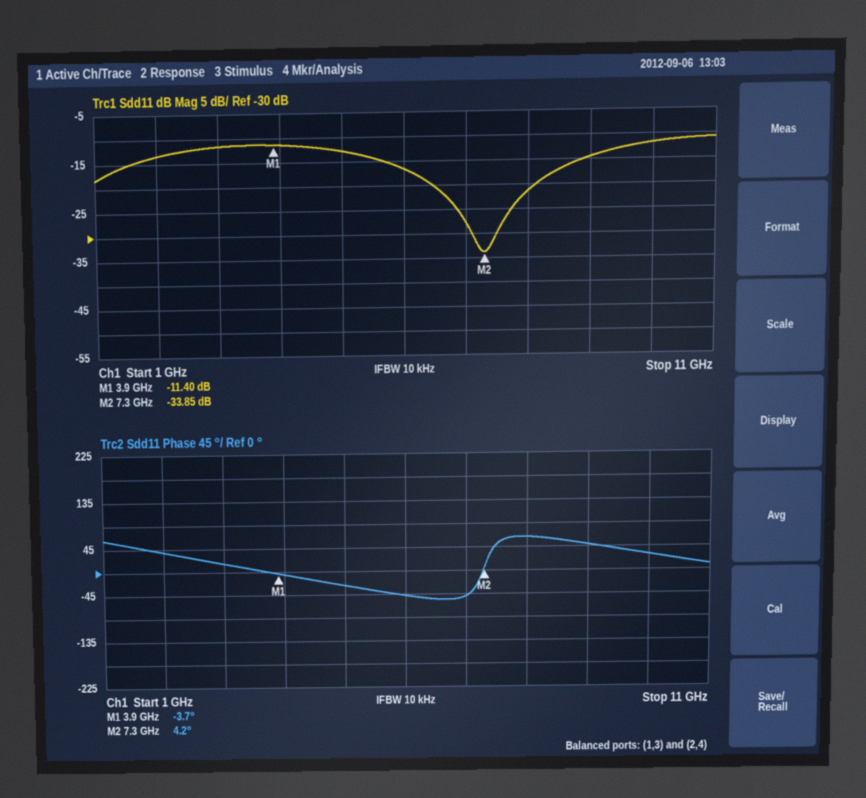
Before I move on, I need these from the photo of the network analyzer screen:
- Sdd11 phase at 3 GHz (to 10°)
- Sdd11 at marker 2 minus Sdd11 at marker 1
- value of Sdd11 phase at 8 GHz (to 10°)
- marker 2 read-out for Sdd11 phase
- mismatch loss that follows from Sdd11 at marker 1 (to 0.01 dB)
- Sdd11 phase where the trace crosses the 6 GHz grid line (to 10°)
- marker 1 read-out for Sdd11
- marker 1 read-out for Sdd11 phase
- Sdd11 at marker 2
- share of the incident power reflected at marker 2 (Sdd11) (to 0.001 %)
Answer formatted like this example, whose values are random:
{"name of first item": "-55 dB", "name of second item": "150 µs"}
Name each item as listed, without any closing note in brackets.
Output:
{"Sdd11 phase at 3 GHz": "20°", "Sdd11 at marker 2 minus Sdd11 at marker 1": "-22.45 dB", "value of Sdd11 phase at 8 GHz": "60°", "marker 2 read-out for Sdd11 phase": "4.2°", "mismatch loss that follows from Sdd11 at marker 1": "0.33 dB", "Sdd11 phase where the trace crosses the 6 GHz grid line": "-50°", "marker 1 read-out for Sdd11": "-11.40 dB", "marker 1 read-out for Sdd11 phase": "-3.7°", "Sdd11 at marker 2": "-33.85 dB", "share of the incident power reflected at marker 2 (Sdd11)": "0.041 %"}
